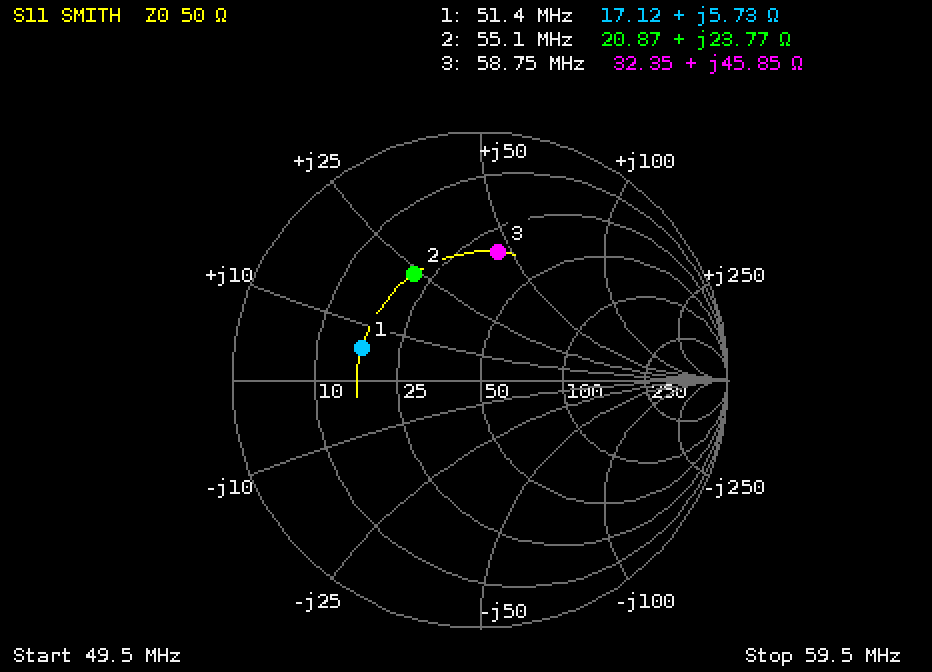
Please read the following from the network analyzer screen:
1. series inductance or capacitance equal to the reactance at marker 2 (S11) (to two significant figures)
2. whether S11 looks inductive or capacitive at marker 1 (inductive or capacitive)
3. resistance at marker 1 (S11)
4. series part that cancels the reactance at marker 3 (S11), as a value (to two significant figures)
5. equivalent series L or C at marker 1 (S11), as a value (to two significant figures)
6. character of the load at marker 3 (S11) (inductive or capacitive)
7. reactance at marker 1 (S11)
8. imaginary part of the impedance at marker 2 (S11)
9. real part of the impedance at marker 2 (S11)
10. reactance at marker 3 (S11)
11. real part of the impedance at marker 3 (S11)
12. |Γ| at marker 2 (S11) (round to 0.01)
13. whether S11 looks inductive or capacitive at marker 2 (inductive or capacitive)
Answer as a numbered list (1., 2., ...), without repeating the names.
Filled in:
1. 69 nH
2. inductive
3. 17.12 Ω
4. 59 pF
5. 18 nH
6. inductive
7. +5.73 Ω
8. +23.77 Ω
9. 20.87 Ω
10. +45.85 Ω
11. 32.35 Ω
12. 0.50
13. inductive
